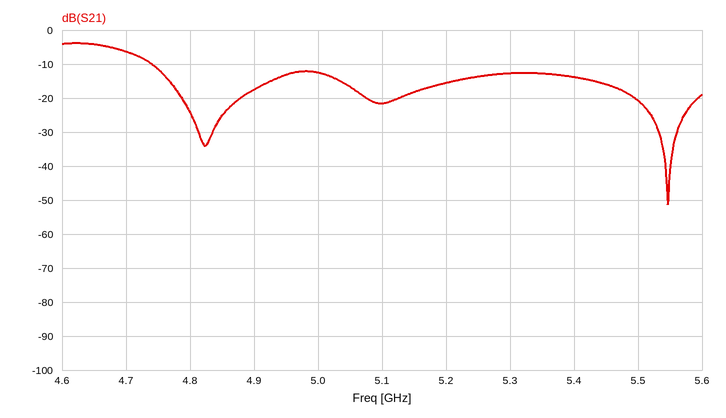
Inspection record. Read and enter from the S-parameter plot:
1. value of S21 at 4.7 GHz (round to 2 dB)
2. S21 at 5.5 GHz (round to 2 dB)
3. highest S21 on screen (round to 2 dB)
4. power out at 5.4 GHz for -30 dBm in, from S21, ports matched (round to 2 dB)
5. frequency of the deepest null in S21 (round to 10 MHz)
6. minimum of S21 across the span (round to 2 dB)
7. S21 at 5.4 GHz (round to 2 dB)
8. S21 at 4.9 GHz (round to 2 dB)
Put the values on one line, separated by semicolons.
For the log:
-6 dB; -20 dB; -4 dB; -44 dBm; 5.55 GHz; -52 dB; -14 dB; -18 dB
